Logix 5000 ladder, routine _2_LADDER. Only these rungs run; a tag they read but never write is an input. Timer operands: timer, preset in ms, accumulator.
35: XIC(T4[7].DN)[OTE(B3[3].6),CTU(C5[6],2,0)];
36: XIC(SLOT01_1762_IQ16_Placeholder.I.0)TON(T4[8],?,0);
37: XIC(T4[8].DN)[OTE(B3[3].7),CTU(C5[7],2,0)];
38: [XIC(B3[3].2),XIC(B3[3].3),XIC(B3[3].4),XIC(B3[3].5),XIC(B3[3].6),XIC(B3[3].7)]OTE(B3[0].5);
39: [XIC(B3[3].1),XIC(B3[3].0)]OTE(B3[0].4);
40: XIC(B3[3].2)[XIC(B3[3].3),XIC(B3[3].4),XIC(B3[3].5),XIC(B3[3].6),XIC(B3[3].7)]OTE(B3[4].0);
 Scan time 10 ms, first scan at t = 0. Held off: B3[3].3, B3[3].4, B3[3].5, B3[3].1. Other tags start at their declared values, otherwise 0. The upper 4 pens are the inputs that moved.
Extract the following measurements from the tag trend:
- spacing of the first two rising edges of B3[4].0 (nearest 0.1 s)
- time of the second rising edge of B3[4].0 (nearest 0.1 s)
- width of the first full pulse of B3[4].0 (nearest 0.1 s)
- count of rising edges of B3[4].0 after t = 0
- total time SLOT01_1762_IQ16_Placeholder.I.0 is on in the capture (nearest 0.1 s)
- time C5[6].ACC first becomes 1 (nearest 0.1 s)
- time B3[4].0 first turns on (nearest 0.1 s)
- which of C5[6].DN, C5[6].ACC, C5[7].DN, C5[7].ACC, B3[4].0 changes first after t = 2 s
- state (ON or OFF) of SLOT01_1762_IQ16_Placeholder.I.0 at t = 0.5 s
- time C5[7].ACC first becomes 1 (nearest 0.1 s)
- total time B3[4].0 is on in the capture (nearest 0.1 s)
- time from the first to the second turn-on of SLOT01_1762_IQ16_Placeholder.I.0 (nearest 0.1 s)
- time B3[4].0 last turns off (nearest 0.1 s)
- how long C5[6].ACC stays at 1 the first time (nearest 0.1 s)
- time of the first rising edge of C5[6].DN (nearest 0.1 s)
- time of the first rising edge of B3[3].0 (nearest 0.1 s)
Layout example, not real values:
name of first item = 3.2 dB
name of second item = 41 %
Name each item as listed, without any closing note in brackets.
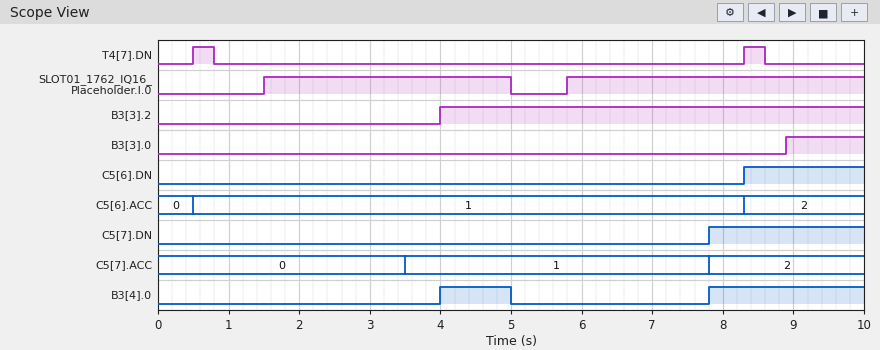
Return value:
spacing of the first two rising edges of B3[4].0 = 3.8 s
time of the second rising edge of B3[4].0 = 7.8 s
width of the first full pulse of B3[4].0 = 1.0 s
count of rising edges of B3[4].0 after t = 0 = 2
total time SLOT01_1762_IQ16_Placeholder.I.0 is on in the capture = 7.7 s
time C5[6].ACC first becomes 1 = 0.5 s
time B3[4].0 first turns on = 4.0 s
which of C5[6].DN, C5[6].ACC, C5[7].DN, C5[7].ACC, B3[4].0 changes first after t = 2 s = C5[7].ACC
state (ON or OFF) of SLOT01_1762_IQ16_Placeholder.I.0 at t = 0.5 s = OFF
time C5[7].ACC first becomes 1 = 3.5 s
total time B3[4].0 is on in the capture = 3.2 s
time from the first to the second turn-on of SLOT01_1762_IQ16_Placeholder.I.0 = 4.3 s
time B3[4].0 last turns off = 5.0 s
how long C5[6].ACC stays at 1 the first time = 7.8 s
time of the first rising edge of C5[6].DN = 8.3 s
time of the first rising edge of B3[3].0 = 8.9 s
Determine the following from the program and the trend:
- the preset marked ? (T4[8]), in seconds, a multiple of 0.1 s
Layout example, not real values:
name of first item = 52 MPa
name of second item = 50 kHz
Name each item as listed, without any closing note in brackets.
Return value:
the preset marked ? (T4[8]), in seconds, a multiple of 0.1 s = 2.0 s
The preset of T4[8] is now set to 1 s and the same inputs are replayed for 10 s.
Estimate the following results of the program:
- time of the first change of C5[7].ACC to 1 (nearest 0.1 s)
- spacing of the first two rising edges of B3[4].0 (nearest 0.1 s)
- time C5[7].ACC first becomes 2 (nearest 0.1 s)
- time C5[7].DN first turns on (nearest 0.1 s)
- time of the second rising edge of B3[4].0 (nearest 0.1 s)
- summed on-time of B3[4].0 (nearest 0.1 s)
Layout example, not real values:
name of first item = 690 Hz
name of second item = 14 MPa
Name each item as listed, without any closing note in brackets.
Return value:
time of the first change of C5[7].ACC to 1 = 2.5 s
spacing of the first two rising edges of B3[4].0 = 2.8 s
time C5[7].ACC first becomes 2 = 6.8 s
time C5[7].DN first turns on = 6.8 s
time of the second rising edge of B3[4].0 = 6.8 s
summed on-time of B3[4].0 = 4.2 s
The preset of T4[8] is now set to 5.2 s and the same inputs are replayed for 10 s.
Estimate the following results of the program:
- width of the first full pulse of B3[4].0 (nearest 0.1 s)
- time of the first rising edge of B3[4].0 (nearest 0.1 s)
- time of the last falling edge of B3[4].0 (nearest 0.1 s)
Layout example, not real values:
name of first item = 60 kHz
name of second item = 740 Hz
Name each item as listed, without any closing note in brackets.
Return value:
width of the first full pulse of B3[4].0 = 0.3 s
time of the first rising edge of B3[4].0 = 8.3 s
time of the last falling edge of B3[4].0 = 8.6 s
